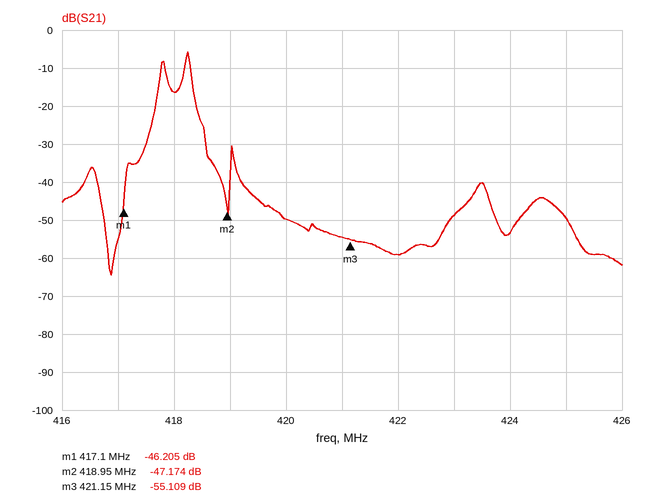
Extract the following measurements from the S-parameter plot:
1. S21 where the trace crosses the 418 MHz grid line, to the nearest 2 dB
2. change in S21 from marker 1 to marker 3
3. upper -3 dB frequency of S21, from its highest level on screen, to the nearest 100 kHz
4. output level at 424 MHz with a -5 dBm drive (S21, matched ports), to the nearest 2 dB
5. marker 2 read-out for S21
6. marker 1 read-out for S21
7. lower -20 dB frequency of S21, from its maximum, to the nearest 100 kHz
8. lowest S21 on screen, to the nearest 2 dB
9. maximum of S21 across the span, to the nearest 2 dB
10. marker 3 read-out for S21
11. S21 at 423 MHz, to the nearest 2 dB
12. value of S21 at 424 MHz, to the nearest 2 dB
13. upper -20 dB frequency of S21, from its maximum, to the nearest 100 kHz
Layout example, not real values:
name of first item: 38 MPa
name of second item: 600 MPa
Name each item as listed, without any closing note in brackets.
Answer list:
S21 where the trace crosses the 418 MHz grid line, to the nearest 2 dB: -16 dB
change in S21 from marker 1 to marker 3: -8.904 dB
upper -3 dB frequency of S21, from its highest level on screen, to the nearest 100 kHz: 418.3 MHz
output level at 424 MHz with a -5 dBm drive (S21, matched ports), to the nearest 2 dB: -58 dBm
marker 2 read-out for S21: -47.174 dB
marker 1 read-out for S21: -46.205 dB
lower -20 dB frequency of S21, from its maximum, to the nearest 100 kHz: 417.6 MHz
lowest S21 on screen, to the nearest 2 dB: -64 dB
maximum of S21 across the span, to the nearest 2 dB: -6 dB
marker 3 read-out for S21: -55.109 dB
S21 at 423 MHz, to the nearest 2 dB: -48 dB
value of S21 at 424 MHz, to the nearest 2 dB: -54 dB
upper -20 dB frequency of S21, from its maximum, to the nearest 100 kHz: 418.5 MHz
